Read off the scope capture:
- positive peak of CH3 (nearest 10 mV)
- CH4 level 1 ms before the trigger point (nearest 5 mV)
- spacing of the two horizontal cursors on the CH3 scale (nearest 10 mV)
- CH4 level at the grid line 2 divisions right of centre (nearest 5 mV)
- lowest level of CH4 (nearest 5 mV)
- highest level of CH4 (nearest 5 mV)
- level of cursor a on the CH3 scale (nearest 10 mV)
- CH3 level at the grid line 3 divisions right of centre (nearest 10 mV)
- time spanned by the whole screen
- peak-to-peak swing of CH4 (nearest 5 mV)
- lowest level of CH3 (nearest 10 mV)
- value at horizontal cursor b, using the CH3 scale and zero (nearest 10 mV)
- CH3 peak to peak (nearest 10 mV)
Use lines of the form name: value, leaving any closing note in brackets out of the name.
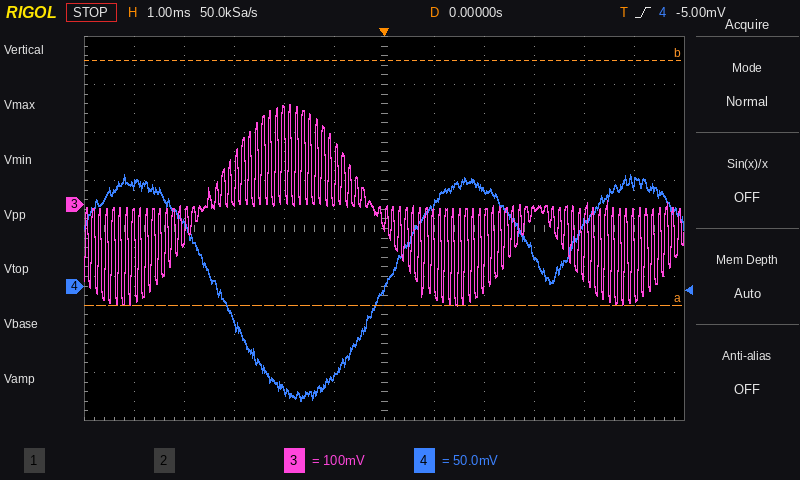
positive peak of CH3: 210 mV
CH4 level 1 ms before the trigger point: -95 mV
spacing of the two horizontal cursors on the CH3 scale: 510 mV
CH4 level at the grid line 2 divisions right of centre: 100 mV
lowest level of CH4: -120 mV
highest level of CH4: 115 mV
level of cursor a on the CH3 scale: -210 mV
CH3 level at the grid line 3 divisions right of centre: -10 mV
time spanned by the whole screen: 12 ms
peak-to-peak swing of CH4: 235 mV
lowest level of CH3: -210 mV
value at horizontal cursor b, using the CH3 scale and zero: 300 mV
CH3 peak to peak: 420 mV
